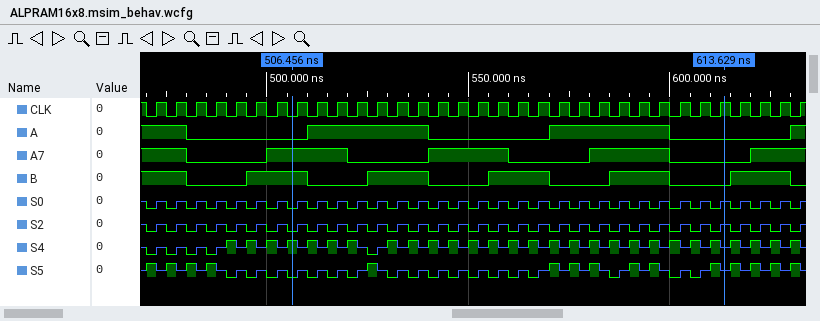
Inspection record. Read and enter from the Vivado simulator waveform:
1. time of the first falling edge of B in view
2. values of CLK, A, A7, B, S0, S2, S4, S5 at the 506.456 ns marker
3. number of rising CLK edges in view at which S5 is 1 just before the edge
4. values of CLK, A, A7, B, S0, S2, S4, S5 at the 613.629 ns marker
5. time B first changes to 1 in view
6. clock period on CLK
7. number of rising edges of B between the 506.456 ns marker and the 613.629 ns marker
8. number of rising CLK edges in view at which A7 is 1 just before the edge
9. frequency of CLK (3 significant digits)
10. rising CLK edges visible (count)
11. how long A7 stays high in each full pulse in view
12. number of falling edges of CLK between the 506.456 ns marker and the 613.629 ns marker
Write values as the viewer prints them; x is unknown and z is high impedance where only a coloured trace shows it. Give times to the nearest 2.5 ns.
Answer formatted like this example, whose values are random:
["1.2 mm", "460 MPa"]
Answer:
["480 ns", "CLK=0, A=0, A7=1, B=1, S0=0, S2=0, S4=1, S5=0", "15", "CLK=1, A=0, A7=0, B=0, S0=z, S2=z, S4=z, S5=z", "495 ns", "5 ns", "3", "17", "200 MHz", "33", "20 ns, 20 ns, 20 ns", "21"]
